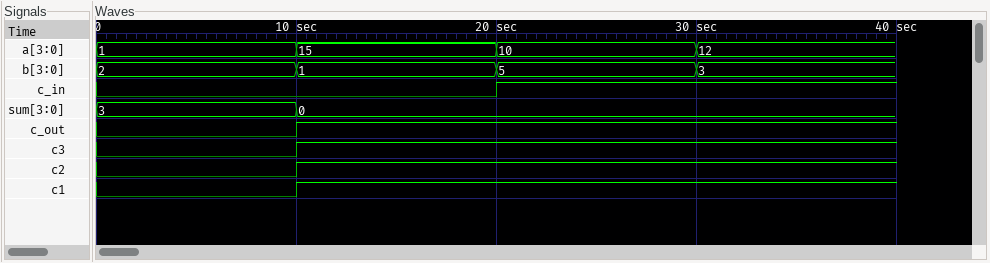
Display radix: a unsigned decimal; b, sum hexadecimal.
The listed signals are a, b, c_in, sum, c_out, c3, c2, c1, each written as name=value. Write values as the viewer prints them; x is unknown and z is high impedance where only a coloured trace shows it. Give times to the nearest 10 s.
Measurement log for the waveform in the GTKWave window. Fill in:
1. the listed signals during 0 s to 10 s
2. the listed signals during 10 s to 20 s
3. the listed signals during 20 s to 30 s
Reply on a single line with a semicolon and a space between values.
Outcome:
a=1, b=2, c_in=0, sum=3, c_out=0, c3=0, c2=0, c1=0; a=15, b=1, c_in=0, sum=0, c_out=1, c3=1, c2=1, c1=1; a=10, b=5, c_in=1, sum=0, c_out=1, c3=1, c2=1, c1=1
